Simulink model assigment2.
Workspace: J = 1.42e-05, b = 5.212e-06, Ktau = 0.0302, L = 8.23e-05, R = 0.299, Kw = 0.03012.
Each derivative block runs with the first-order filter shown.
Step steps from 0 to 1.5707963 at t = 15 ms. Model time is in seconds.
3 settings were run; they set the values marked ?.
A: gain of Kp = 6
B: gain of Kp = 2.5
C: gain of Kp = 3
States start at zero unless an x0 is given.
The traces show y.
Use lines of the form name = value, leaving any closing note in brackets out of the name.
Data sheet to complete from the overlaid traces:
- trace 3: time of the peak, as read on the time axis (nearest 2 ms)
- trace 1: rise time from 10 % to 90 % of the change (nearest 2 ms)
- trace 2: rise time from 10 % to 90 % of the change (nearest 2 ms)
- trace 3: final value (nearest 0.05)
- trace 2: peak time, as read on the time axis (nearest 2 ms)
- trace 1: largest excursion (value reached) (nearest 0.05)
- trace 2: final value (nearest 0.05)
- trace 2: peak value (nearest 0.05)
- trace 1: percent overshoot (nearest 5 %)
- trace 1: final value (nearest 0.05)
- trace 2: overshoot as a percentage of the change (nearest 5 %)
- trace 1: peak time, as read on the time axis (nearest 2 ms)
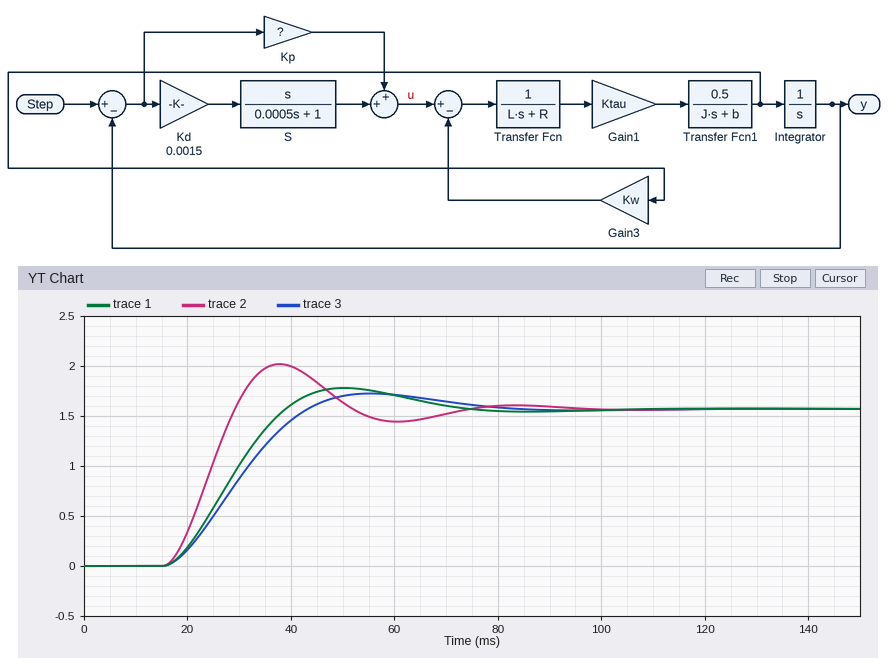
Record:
trace 3: time of the peak, as read on the time axis = 56 ms
trace 1: rise time from 10 % to 90 % of the change = 16 ms
trace 2: rise time from 10 % to 90 % of the change = 10 ms
trace 3: final value = 1.55
trace 2: peak time, as read on the time axis = 38 ms
trace 1: largest excursion (value reached) = 1.80
trace 2: final value = 1.55
trace 2: peak value = 2.00
trace 1: percent overshoot = 15 %
trace 1: final value = 1.55
trace 2: overshoot as a percentage of the change = 30 %
trace 1: peak time, as read on the time axis = 50 ms
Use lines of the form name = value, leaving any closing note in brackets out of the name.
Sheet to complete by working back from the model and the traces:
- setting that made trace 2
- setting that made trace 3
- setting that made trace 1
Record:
setting that made trace 2 = A
setting that made trace 3 = B
setting that made trace 1 = C
